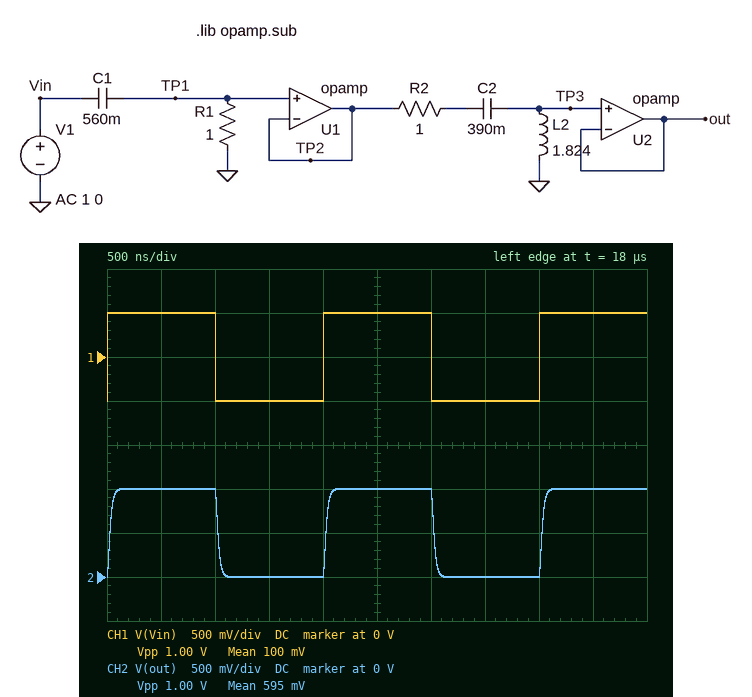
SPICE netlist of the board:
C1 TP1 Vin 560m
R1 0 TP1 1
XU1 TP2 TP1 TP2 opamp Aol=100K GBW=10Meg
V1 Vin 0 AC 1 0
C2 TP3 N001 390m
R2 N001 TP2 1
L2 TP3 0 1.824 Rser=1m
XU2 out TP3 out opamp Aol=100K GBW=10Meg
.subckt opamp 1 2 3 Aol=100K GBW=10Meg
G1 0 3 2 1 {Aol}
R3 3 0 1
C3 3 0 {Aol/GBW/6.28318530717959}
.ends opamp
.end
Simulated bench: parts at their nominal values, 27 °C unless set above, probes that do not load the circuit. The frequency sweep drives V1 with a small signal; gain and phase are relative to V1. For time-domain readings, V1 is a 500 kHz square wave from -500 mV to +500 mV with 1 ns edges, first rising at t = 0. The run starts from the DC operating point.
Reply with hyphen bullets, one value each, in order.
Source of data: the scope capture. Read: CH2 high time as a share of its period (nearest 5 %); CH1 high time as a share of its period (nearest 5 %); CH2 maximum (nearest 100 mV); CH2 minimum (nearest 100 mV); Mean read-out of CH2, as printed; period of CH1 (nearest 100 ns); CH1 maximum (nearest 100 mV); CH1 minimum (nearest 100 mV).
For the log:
- 50 %
- 50 %
- 1.0 V
- 0 V
- 595 mV
- 2.0 µs
- 500 mV
- -500 mV
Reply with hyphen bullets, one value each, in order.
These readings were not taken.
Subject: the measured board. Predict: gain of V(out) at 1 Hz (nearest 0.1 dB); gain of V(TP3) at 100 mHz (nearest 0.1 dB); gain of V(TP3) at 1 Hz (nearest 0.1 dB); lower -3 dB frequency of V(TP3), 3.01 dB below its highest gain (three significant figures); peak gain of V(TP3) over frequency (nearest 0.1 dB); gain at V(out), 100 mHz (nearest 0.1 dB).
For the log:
- -0.1 dB
- -18.2 dB
- -0.1 dB
- 170 mHz
- 2.3 dB
- -18.2 dB
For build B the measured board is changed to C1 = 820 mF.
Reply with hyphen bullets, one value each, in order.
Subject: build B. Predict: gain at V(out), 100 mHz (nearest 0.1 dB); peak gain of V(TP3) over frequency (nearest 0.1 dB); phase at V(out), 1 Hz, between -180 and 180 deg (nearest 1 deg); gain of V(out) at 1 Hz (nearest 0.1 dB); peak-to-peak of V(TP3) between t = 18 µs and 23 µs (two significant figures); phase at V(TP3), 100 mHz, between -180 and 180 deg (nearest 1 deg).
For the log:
- -15.4 dB
- 4.1 dB
- 16 deg
- 0.1 dB
- 1.0 V
- -136 deg
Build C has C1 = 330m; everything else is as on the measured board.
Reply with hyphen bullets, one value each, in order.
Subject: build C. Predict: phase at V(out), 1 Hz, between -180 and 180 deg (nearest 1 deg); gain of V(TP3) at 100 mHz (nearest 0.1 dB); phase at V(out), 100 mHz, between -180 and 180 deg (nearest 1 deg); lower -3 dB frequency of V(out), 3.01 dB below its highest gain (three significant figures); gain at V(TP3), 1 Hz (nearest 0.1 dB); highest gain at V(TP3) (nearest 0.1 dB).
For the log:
- 31 deg
- -22.5 dB
- -121 deg
- 180 mHz
- -0.6 dB
- 0 dB
